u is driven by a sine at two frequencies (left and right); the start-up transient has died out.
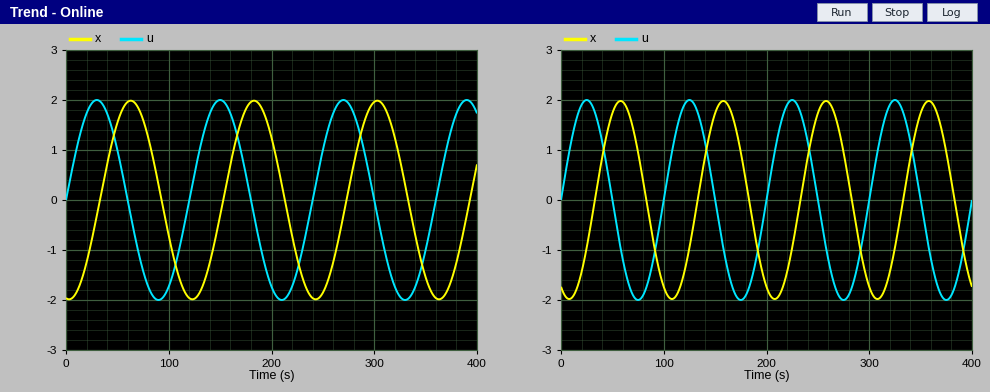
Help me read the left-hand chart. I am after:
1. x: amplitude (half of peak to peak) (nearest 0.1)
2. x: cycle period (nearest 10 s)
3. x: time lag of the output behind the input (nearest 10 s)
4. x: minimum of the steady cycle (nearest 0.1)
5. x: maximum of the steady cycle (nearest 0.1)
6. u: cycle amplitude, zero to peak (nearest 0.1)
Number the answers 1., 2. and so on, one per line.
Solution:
1. 2.0
2. 120 s
3. 30 s
4. -2.0
5. 2.0
6. 2.0
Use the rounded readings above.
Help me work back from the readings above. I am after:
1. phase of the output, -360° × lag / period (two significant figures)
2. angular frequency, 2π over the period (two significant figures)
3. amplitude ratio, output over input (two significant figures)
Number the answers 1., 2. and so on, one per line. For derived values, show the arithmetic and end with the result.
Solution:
1. -360 × 30 / 120 = -90°
2. 2π / 120 = 0.052 rad/s
3. 2 / 2 = 1.0
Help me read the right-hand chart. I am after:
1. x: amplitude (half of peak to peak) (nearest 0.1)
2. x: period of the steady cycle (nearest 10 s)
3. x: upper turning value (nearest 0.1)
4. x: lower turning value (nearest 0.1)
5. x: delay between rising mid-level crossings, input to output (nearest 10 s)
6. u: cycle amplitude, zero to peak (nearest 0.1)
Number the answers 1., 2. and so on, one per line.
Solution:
1. 2.0
2. 100 s
3. 2.0
4. -2.0
5. 30 s
6. 2.0
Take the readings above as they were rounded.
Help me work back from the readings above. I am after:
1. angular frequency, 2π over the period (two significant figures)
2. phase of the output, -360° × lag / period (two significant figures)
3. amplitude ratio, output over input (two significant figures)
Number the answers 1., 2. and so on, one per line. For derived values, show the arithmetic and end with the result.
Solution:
1. 2π / 100 = 0.063 rad/s
2. -360 × 30 / 100 = -110°
3. 2 / 2 = 1.0
